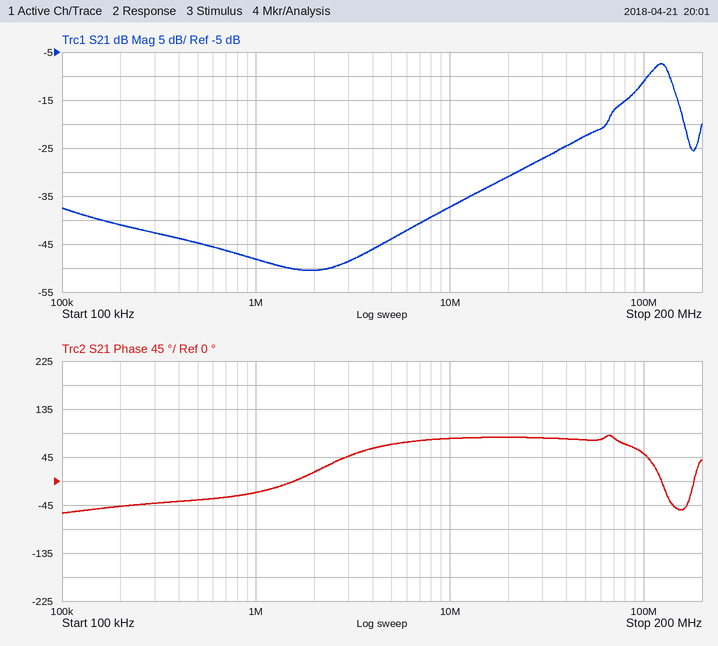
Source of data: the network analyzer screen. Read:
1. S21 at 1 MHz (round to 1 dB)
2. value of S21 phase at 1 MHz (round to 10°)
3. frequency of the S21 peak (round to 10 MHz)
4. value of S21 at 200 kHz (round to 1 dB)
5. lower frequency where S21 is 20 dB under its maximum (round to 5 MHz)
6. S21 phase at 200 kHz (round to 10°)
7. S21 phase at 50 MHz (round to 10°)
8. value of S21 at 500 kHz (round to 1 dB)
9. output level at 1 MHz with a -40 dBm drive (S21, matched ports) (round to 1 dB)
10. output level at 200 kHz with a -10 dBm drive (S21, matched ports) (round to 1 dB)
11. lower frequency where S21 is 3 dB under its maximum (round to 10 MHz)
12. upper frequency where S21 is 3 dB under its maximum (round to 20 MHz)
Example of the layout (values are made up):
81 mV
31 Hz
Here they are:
-48 dB
-20°
120 MHz
-41 dB
30 MHz
-50°
80°
-45 dB
-88 dBm
-51 dBm
100 MHz
140 MHz
